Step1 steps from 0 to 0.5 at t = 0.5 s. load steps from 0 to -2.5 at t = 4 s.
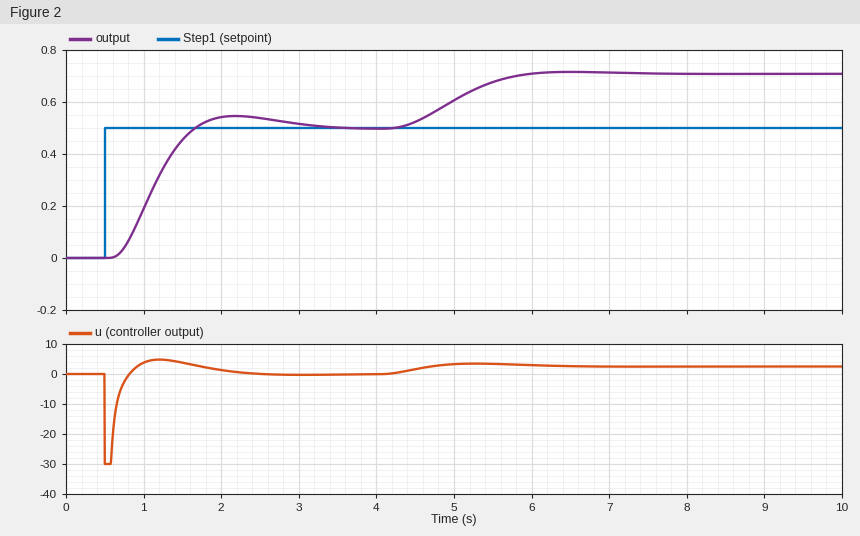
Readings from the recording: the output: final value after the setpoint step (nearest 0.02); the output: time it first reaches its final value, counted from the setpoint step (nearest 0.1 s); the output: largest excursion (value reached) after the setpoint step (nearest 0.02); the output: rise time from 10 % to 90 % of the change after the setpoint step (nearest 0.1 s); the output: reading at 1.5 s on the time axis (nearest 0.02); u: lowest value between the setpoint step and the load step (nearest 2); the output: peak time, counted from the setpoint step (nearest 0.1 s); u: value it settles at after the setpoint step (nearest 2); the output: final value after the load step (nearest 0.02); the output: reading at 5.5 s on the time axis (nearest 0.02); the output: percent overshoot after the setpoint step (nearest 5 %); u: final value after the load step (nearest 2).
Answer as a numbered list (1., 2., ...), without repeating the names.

1. 0.50
2. 1.2 s
3. 0.54
4. 0.7 s
5. 0.46
6. -30
7. 1.7 s
8. 0
9. 0.70
10. 0.68
11. 10 %
12. 2
